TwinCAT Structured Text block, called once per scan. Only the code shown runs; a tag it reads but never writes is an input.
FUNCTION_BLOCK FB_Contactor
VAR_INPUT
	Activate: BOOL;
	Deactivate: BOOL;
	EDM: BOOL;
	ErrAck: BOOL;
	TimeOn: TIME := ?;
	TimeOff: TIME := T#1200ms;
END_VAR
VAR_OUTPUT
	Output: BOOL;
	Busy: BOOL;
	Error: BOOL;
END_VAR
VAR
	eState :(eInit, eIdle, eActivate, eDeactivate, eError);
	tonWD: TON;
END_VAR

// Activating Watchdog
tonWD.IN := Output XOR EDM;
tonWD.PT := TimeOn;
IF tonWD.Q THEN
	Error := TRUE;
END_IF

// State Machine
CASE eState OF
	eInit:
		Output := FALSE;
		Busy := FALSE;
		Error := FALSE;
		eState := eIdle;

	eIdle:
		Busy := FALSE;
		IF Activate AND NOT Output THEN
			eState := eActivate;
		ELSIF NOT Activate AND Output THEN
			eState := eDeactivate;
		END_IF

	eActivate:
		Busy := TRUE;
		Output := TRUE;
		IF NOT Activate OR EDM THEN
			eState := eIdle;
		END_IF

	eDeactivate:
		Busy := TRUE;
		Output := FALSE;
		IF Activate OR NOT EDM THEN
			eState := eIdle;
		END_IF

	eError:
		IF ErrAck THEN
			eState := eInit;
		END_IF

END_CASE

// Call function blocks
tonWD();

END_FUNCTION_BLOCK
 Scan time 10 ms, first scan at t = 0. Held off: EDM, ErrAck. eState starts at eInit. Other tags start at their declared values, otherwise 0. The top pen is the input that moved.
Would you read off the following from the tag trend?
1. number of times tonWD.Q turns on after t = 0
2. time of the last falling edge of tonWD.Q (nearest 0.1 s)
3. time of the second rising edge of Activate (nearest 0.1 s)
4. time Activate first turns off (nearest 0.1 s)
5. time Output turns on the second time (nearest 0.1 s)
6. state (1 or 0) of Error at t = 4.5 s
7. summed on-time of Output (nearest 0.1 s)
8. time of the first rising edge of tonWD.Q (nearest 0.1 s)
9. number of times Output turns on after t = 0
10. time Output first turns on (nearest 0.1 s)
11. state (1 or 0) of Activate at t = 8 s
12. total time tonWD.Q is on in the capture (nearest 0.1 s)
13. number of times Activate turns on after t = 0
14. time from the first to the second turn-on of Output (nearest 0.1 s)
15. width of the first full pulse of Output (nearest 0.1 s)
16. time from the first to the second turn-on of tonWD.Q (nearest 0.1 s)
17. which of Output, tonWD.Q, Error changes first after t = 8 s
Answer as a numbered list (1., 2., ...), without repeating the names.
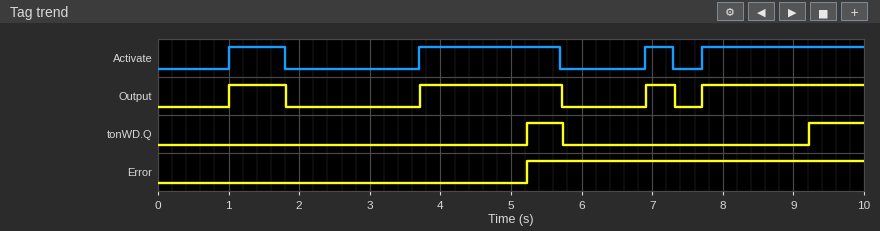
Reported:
1. 2
2. 5.7 s
3. 3.7 s
4. 1.8 s
5. 3.7 s
6. 0
7. 5.5 s
8. 5.2 s
9. 4
10. 1.0 s
11. 1
12. 1.3 s
13. 4
14. 2.7 s
15. 0.8 s
16. 4.0 s
17. tonWD.Q
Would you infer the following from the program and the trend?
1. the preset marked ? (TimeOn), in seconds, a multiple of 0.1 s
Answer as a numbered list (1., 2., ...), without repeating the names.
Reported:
1. 1.5 s
